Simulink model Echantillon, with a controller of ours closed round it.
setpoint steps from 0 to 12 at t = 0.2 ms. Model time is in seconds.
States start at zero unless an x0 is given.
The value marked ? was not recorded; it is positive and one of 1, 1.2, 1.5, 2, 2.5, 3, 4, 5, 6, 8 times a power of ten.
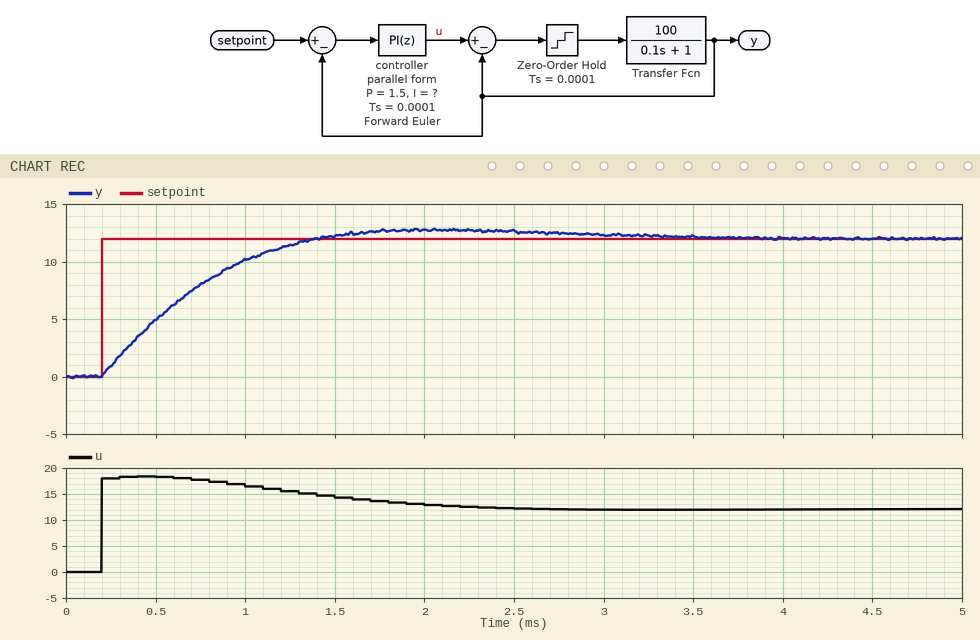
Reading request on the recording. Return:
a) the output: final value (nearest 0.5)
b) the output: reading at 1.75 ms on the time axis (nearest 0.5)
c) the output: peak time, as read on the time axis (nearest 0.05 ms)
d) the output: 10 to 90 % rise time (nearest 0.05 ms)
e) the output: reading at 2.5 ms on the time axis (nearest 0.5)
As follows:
12.0
12.5
2.10 ms
0.85 ms
12.5
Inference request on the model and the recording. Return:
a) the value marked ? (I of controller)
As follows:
2500
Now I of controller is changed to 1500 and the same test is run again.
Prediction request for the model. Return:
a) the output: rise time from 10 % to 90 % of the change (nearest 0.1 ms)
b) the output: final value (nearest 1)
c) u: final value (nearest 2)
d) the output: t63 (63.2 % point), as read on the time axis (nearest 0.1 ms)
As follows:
1.4 ms
12
12
0.8 ms
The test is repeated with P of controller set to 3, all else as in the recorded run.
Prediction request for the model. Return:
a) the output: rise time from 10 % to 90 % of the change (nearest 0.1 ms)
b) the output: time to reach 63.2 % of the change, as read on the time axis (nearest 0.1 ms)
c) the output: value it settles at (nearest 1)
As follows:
0.7 ms
0.5 ms
12
